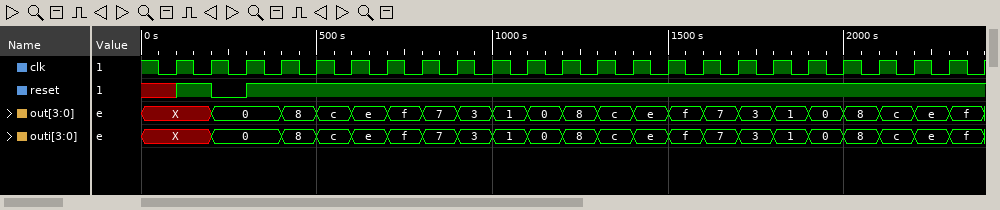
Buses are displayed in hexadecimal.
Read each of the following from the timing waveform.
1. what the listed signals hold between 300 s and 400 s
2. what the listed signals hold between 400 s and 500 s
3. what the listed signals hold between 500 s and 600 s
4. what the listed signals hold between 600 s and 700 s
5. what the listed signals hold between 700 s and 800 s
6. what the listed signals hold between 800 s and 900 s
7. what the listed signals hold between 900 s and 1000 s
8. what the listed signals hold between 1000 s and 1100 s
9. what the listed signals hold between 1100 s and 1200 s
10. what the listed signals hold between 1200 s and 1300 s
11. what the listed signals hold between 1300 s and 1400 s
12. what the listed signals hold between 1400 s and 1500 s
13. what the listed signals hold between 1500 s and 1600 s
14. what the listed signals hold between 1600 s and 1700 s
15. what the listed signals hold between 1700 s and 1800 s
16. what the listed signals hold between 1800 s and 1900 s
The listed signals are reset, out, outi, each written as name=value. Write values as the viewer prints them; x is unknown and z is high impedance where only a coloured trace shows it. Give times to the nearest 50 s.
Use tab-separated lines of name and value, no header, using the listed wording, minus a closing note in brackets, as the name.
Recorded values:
what the listed signals hold between 300 s and 400 s	reset=1, out=0, outi=0
what the listed signals hold between 400 s and 500 s	reset=1, out=8, outi=8
what the listed signals hold between 500 s and 600 s	reset=1, out=c, outi=c
what the listed signals hold between 600 s and 700 s	reset=1, out=e, outi=e
what the listed signals hold between 700 s and 800 s	reset=1, out=f, outi=f
what the listed signals hold between 800 s and 900 s	reset=1, out=7, outi=7
what the listed signals hold between 900 s and 1000 s	reset=1, out=3, outi=3
what the listed signals hold between 1000 s and 1100 s	reset=1, out=1, outi=1
what the listed signals hold between 1100 s and 1200 s	reset=1, out=0, outi=0
what the listed signals hold between 1200 s and 1300 s	reset=1, out=8, outi=8
what the listed signals hold between 1300 s and 1400 s	reset=1, out=c, outi=c
what the listed signals hold between 1400 s and 1500 s	reset=1, out=e, outi=e
what the listed signals hold between 1500 s and 1600 s	reset=1, out=f, outi=f
what the listed signals hold between 1600 s and 1700 s	reset=1, out=7, outi=7
what the listed signals hold between 1700 s and 1800 s	reset=1, out=3, outi=3
what the listed signals hold between 1800 s and 1900 s	reset=1, out=1, outi=1
